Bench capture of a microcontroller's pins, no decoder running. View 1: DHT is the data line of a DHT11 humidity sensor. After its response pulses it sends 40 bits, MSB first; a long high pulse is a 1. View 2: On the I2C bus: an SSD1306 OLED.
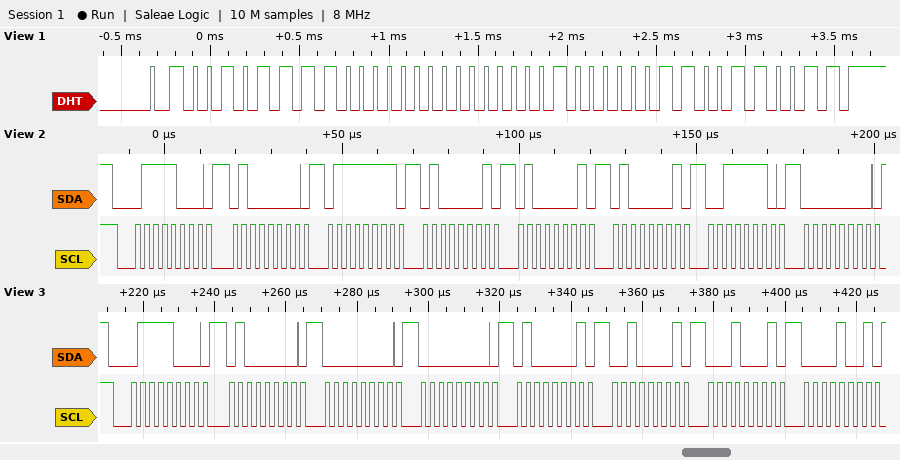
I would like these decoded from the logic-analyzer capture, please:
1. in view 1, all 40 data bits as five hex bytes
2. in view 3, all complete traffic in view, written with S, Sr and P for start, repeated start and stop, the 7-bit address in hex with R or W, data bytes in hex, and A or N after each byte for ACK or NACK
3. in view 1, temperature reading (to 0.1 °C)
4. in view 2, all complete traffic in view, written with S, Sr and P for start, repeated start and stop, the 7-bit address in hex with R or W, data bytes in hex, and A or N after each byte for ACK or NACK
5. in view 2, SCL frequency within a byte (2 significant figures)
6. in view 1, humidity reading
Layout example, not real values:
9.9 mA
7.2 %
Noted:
2F 00 01 03 33
S 3CW A 40 A 00 A 00 A 41 A 21 A 11 A 09 A
1.3 °C
S 3CW A 40 A 7F A 41 A 41 A 41 A 3E A 00 A
400 kHz
47 %
